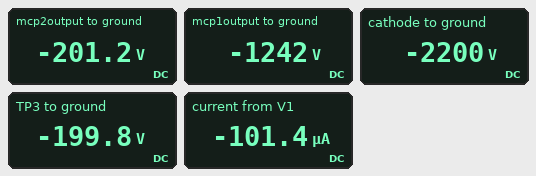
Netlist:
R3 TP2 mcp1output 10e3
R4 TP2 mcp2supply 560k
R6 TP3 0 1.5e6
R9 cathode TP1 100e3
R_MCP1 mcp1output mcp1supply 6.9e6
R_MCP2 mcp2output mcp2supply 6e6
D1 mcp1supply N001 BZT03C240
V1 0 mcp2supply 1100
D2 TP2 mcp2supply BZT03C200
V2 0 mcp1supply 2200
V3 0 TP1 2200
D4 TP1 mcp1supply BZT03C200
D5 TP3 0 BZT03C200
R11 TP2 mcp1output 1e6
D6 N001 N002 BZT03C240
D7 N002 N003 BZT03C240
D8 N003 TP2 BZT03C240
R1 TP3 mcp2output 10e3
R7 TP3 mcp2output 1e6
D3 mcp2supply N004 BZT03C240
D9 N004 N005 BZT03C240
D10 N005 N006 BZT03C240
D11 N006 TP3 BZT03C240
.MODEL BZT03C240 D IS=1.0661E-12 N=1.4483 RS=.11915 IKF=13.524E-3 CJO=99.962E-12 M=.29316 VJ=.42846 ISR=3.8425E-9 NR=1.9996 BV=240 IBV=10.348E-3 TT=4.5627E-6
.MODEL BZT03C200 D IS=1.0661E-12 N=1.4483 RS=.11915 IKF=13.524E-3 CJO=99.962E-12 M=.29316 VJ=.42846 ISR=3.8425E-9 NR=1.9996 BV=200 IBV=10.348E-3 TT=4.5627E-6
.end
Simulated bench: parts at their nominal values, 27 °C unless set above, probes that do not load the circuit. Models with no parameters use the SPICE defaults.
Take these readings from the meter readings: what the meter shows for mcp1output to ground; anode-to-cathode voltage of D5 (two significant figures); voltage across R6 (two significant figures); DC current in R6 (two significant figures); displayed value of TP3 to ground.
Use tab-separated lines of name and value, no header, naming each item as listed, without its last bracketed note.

what the meter shows for mcp1output to ground	-1242 V
anode-to-cathode voltage of D5	-200 V
voltage across R6	200 V
DC current in R6	130 µA
displayed value of TP3 to ground	-199.8 V
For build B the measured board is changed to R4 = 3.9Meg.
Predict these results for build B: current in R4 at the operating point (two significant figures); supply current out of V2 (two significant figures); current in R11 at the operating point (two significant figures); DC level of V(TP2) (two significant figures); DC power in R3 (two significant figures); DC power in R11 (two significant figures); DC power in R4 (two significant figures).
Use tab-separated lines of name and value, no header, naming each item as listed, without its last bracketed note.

current in R4 at the operating point	51 µA
supply current out of V2	130 µA
current in R11 at the operating point	1.3 µA
DC level of V(TP2)	-1.3 kV
DC power in R3	170 µW
DC power in R11	1.7 µW
DC power in R4	10 mW
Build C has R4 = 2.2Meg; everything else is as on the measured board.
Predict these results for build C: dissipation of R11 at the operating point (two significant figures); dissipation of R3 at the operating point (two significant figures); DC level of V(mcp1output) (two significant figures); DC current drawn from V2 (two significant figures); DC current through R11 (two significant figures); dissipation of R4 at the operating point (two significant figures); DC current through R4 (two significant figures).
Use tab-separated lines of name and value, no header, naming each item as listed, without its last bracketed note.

dissipation of R11 at the operating point	1.7 µW
dissipation of R3 at the operating point	170 µW
DC level of V(mcp1output)	-1.3 kV
DC current drawn from V2	130 µA
DC current through R11	1.3 µA
dissipation of R4 at the operating point	18 mW
DC current through R4	91 µA
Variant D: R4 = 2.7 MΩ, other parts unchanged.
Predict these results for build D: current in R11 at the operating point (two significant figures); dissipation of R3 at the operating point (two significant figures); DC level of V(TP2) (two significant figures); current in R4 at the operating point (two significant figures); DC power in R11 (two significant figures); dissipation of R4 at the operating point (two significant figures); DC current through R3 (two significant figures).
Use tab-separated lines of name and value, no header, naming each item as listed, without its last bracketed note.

current in R11 at the operating point	1.3 µA
dissipation of R3 at the operating point	170 µW
DC level of V(TP2)	-1.3 kV
current in R4 at the operating point	74 µA
DC power in R11	1.7 µW
dissipation of R4 at the operating point	15 mW
DC current through R3	130 µA
